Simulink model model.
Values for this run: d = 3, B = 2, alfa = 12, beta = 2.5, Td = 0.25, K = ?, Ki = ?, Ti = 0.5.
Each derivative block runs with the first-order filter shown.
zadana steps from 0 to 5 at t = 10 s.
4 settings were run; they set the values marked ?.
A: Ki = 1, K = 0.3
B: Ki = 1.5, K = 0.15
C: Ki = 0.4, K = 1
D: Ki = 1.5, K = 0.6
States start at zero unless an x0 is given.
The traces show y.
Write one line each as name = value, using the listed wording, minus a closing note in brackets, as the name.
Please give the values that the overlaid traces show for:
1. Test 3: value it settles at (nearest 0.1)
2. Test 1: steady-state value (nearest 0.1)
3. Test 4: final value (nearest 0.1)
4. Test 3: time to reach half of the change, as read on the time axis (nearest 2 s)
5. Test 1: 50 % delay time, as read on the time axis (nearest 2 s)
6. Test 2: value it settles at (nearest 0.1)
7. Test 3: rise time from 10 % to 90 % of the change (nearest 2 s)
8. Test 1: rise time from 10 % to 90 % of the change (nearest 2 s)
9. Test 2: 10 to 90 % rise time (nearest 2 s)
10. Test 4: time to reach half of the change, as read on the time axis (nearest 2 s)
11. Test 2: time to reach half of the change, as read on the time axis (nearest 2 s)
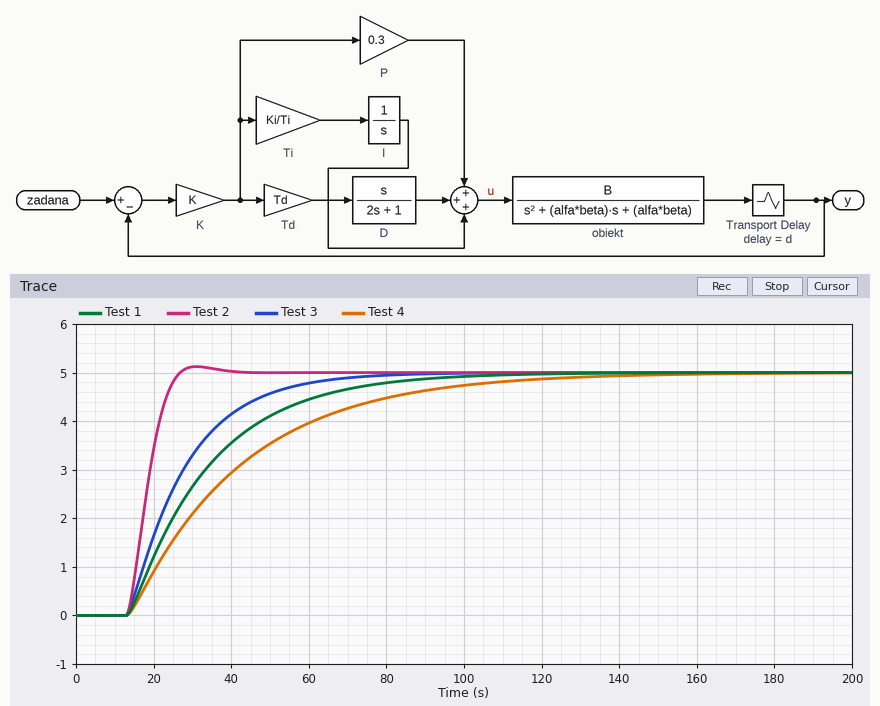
Test 3: value it settles at = 5.0
Test 1: steady-state value = 5.0
Test 4: final value = 5.0
Test 3: time to reach half of the change, as read on the time axis = 24 s
Test 1: 50 % delay time, as read on the time axis = 28 s
Test 2: value it settles at = 5.0
Test 3: rise time from 10 % to 90 % of the change = 32 s
Test 1: rise time from 10 % to 90 % of the change = 46 s
Test 2: 10 to 90 % rise time = 8 s
Test 4: time to reach half of the change, as read on the time axis = 34 s
Test 2: time to reach half of the change, as read on the time axis = 18 s
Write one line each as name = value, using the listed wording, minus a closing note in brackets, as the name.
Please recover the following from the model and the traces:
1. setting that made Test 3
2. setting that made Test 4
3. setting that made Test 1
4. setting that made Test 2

setting that made Test 3 = C
setting that made Test 4 = B
setting that made Test 1 = A
setting that made Test 2 = D
